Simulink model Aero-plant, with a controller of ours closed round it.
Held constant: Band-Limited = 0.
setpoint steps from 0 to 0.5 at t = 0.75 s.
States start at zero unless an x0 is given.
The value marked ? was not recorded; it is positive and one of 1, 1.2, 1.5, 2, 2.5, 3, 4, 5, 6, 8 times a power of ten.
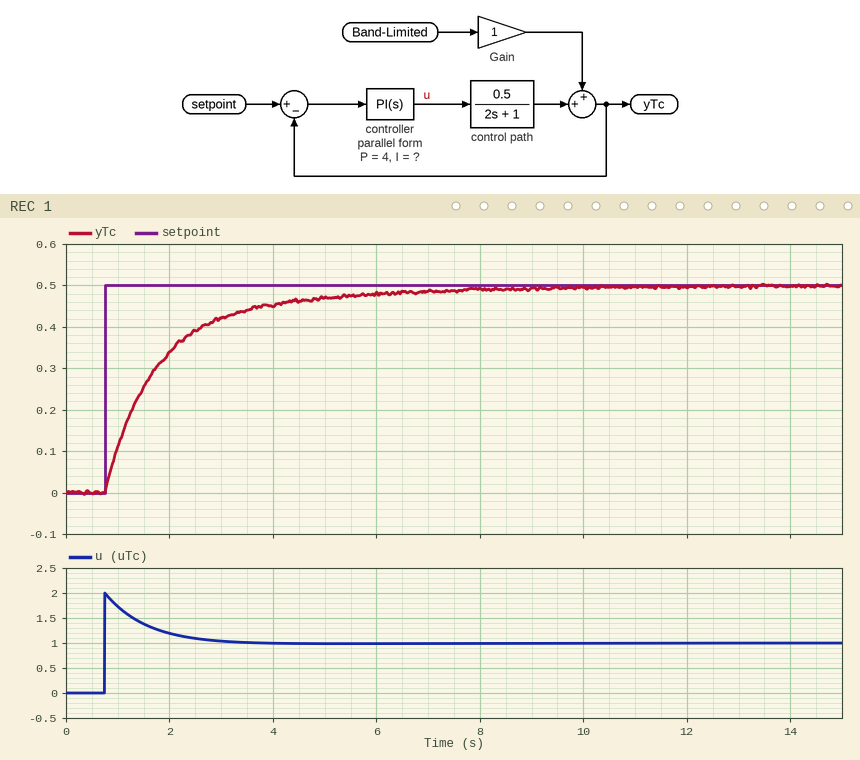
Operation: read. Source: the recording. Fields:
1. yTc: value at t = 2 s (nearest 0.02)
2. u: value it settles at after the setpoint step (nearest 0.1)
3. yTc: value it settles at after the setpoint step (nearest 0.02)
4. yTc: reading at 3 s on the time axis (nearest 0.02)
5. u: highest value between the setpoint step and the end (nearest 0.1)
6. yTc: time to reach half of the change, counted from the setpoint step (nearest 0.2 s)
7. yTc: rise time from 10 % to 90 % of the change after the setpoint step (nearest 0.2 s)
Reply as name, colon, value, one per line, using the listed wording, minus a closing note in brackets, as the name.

yTc: value at t = 2 s: 0.34
u: value it settles at after the setpoint step: 1.0
yTc: value it settles at after the setpoint step: 0.50
yTc: reading at 3 s on the time axis: 0.42
u: highest value between the setpoint step and the end: 2.0
yTc: time to reach half of the change, counted from the setpoint step: 0.8 s
yTc: rise time from 10 % to 90 % of the change after the setpoint step: 3.0 s
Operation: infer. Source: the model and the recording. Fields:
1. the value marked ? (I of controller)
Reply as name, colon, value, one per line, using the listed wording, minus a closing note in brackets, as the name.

the value marked ?: 1.5
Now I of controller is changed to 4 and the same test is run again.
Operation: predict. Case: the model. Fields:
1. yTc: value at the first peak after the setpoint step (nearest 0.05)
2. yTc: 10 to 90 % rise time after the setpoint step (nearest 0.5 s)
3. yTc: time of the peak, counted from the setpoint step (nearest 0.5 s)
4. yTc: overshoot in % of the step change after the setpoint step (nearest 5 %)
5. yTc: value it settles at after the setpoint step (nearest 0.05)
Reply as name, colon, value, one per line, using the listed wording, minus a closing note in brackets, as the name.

yTc: value at the first peak after the setpoint step: 0.55
yTc: 10 to 90 % rise time after the setpoint step: 1.5 s
yTc: time of the peak, counted from the setpoint step: 3.0 s
yTc: overshoot in % of the step change after the setpoint step: 10 %
yTc: value it settles at after the setpoint step: 0.50
